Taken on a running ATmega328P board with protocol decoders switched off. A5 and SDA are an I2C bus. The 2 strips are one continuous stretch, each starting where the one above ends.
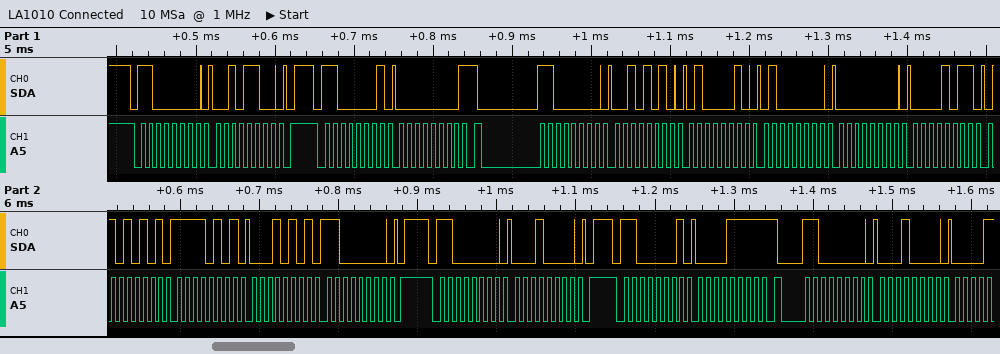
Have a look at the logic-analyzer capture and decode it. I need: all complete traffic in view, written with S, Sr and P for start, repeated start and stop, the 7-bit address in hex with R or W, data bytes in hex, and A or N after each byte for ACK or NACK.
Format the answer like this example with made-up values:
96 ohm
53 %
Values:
S 60W A 2C A P S 60R A 00 N Sr 60W A 2A A 42 A 40 A 00 A 0B A 55 A F5 A 15 A C0 A P S 60W A 10 A P S 60R A 0F N Sr 60W A 10 A
